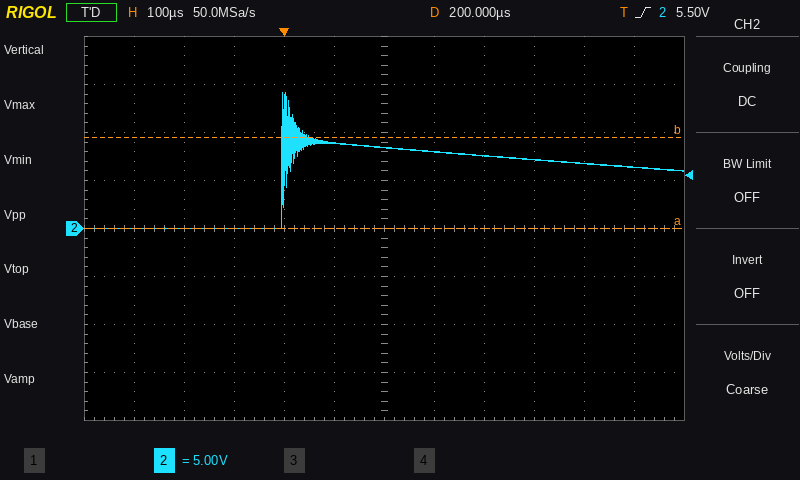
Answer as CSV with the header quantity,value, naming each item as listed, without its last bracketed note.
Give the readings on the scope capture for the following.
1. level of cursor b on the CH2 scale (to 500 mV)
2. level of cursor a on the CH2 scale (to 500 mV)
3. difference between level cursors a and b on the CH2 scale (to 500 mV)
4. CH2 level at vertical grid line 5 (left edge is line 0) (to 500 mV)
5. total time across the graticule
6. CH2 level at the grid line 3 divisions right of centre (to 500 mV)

quantity,value
level of cursor b on the CH2 scale,9.5 V
level of cursor a on the CH2 scale,0.0 V
difference between level cursors a and b on the CH2 scale,9.5 V
CH2 level at vertical grid line 5 (left edge is line 0),9.0 V
total time across the graticule,1.2 ms
CH2 level at the grid line 3 divisions right of centre,7.0 V
